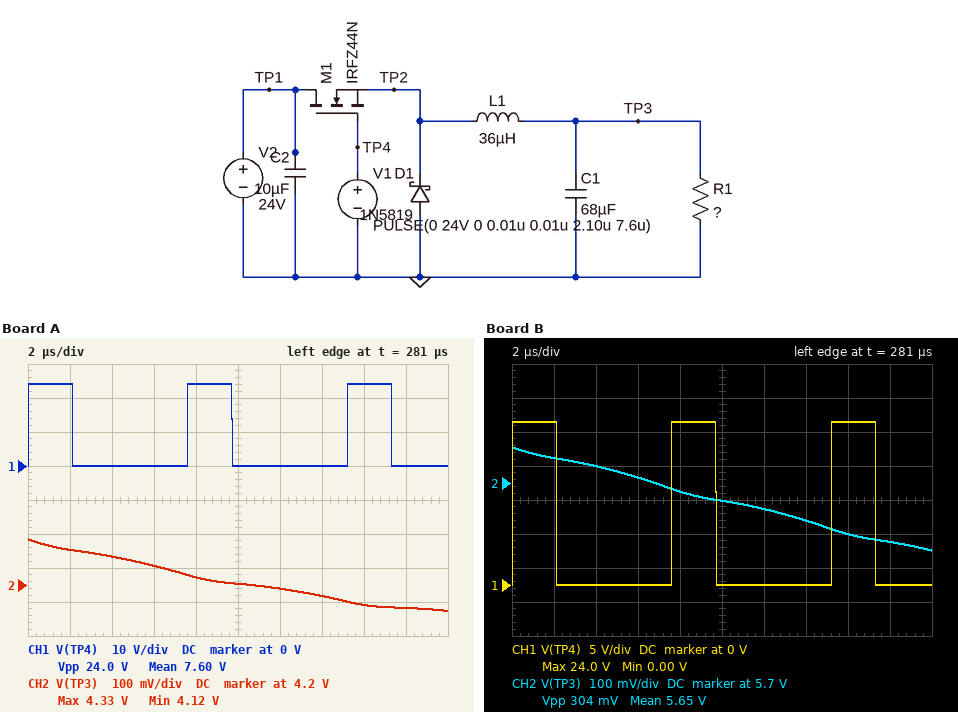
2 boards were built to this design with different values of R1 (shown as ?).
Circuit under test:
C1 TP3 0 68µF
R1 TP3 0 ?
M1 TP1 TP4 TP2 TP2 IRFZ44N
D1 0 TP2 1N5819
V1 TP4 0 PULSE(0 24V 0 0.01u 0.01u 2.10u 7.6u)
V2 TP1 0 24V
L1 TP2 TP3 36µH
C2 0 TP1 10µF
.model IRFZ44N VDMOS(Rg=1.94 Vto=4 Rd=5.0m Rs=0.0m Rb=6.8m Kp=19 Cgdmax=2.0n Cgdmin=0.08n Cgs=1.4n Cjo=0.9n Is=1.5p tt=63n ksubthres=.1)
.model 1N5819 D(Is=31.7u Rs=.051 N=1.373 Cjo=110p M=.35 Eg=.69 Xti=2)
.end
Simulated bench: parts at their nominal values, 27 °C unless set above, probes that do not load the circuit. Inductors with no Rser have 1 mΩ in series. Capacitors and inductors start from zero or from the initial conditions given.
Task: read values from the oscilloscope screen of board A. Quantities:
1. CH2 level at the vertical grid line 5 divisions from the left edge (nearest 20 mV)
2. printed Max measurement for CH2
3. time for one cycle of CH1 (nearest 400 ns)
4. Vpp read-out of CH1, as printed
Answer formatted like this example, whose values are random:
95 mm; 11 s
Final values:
4.20 V; 4.33 V; 7.6 µs; 24.0 V
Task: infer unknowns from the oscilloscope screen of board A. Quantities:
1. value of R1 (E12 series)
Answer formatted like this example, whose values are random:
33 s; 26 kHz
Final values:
2.2 Ω
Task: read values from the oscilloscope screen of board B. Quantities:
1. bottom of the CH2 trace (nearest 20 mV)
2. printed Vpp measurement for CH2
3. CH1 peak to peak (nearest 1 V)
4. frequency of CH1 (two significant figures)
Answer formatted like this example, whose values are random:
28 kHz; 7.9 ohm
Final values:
5.50 V; 304 mV; 24 V; 130 kHz
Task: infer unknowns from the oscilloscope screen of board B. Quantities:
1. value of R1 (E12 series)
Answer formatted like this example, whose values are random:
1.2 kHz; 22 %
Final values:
3.9 Ω
